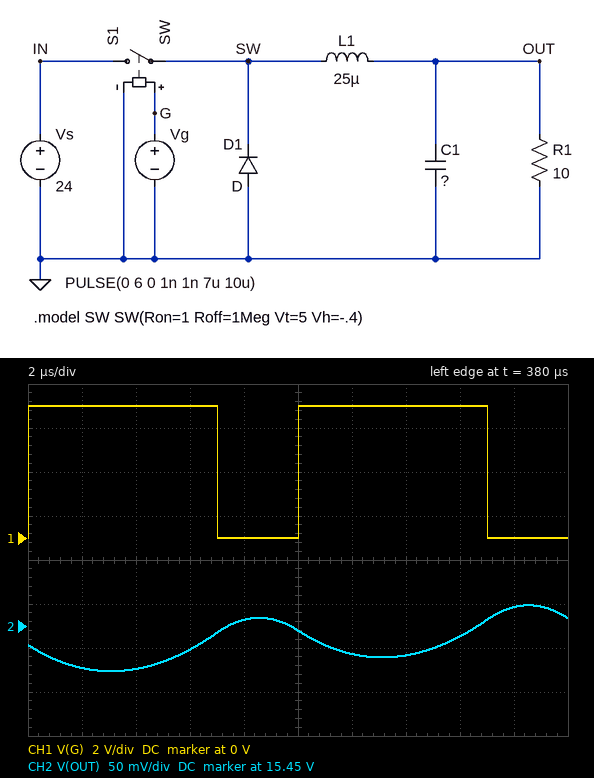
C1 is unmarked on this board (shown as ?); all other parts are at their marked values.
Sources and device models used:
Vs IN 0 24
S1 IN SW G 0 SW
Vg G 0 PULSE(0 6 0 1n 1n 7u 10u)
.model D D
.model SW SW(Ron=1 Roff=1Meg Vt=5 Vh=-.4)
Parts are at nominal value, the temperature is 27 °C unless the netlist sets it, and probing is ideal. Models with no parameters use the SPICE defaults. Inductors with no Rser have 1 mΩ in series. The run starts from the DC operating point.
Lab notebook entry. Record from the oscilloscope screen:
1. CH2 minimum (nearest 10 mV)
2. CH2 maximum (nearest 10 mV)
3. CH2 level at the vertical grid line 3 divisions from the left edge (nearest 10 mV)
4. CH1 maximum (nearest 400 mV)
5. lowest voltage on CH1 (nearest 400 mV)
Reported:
15.40 V
15.47 V
15.42 V
6.0 V
0 V
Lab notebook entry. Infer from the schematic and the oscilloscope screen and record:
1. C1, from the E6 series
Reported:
47 µF
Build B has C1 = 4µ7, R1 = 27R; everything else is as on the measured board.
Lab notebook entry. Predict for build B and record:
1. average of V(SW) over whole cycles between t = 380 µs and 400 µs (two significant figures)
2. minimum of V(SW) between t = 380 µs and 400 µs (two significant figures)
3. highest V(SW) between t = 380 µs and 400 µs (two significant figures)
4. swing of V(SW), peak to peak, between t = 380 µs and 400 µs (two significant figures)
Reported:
18 V
-840 mV
24 V
25 V
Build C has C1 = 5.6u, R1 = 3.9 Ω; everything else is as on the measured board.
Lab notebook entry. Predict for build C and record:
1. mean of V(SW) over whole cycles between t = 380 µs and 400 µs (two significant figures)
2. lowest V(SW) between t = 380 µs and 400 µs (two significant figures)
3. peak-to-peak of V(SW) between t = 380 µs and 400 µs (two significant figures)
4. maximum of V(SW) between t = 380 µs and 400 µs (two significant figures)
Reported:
14 V
-870 mV
22 V
21 V
